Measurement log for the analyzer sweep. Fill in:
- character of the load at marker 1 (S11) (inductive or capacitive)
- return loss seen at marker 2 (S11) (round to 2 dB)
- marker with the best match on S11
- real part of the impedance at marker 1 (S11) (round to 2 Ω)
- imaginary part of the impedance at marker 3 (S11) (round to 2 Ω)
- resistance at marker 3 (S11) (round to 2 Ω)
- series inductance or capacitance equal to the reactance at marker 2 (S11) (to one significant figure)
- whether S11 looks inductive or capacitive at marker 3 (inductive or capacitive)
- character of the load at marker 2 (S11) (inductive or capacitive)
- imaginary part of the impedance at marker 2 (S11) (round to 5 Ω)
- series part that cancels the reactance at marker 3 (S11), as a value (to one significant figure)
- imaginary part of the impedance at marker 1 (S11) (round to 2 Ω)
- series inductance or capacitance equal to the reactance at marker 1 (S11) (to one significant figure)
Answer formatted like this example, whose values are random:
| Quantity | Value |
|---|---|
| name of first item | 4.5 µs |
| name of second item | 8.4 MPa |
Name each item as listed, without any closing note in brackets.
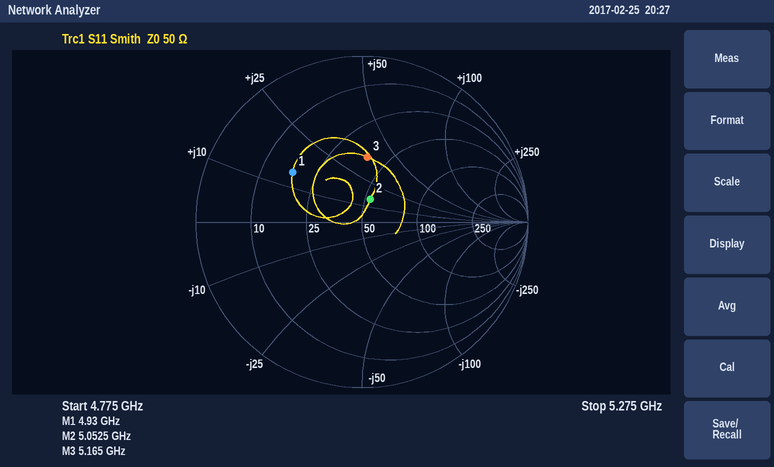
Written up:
| Quantity | Value |
|---|---|
| character of the load at marker 1 (S11) | inductive |
| return loss seen at marker 2 (S11) | 16 dB |
| marker with the best match on S11 | marker 2 |
| real part of the impedance at marker 1 (S11) | 18 Ω |
| imaginary part of the impedance at marker 3 (S11) | +36 Ω |
| resistance at marker 3 (S11) | 38 Ω |
| series inductance or capacitance equal to the reactance at marker 2 (S11) | 500 pH |
| whether S11 looks inductive or capacitive at marker 3 | inductive |
| character of the load at marker 2 (S11) | inductive |
| imaginary part of the impedance at marker 2 (S11) | +15 Ω |
| series part that cancels the reactance at marker 3 (S11), as a value | 900 fF |
| imaginary part of the impedance at marker 1 (S11) | +14 Ω |
| series inductance or capacitance equal to the reactance at marker 1 (S11) | 500 pH |
